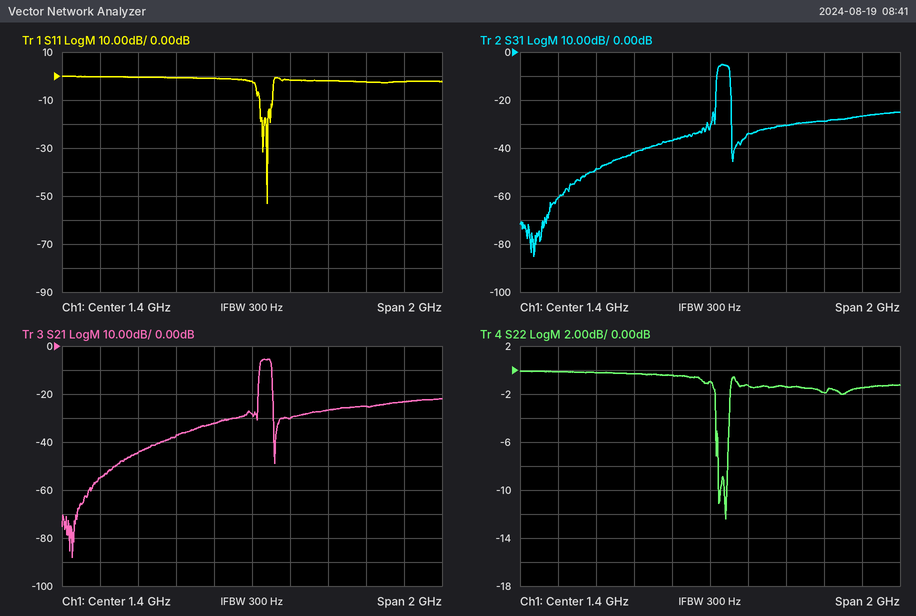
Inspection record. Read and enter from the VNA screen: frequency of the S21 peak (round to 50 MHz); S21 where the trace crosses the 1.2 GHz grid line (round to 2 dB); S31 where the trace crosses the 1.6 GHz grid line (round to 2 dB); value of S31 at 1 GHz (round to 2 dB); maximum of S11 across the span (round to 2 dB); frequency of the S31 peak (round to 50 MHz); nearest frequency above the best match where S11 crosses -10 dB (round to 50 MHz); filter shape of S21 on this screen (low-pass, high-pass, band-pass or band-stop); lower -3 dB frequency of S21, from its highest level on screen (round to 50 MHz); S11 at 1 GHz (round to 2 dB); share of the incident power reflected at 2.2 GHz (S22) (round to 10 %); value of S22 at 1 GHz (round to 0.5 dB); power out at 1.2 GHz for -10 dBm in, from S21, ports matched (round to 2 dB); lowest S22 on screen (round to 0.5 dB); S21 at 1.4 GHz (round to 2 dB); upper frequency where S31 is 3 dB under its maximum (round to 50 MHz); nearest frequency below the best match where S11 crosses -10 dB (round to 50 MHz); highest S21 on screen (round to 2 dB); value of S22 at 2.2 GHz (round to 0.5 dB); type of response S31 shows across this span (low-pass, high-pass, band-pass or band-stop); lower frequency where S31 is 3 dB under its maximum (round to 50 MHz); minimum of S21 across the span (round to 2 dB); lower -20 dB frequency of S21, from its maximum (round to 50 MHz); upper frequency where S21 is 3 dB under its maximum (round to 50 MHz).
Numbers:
1.45 GHz
-32 dB
-34 dB
-42 dB
0 dB
1.45 GHz
1.50 GHz
band-pass
1.45 GHz
0 dB
70 %
-0.5 dB
-42 dBm
-12.5 dB
-28 dB
1.50 GHz
1.45 GHz
-6 dB
-1.5 dB
band-pass
1.45 GHz
-88 dB
1.45 GHz
1.50 GHz
